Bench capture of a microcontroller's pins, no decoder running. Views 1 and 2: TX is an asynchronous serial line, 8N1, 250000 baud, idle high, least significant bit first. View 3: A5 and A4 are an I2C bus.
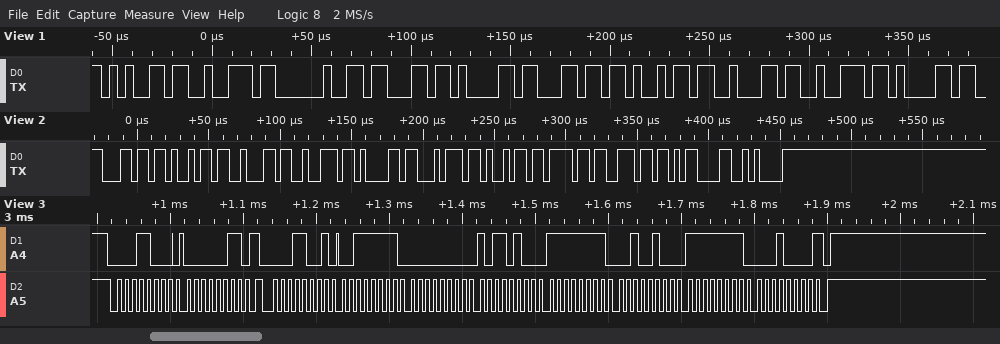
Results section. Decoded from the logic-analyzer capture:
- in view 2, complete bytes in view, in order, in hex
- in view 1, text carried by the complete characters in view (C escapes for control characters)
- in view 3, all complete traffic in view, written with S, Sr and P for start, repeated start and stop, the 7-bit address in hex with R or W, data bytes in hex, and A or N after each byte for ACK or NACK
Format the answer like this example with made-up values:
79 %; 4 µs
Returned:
0x6C 0x69 0x62 0x72 0x61 0x74 0x69 0x6F 0x6E 0x0D 0x0A; "er calibra"; S 0CW A 03 A Sr 0CR A 3F A 00 A B4 A FF A 24 A FF A 10 N P
